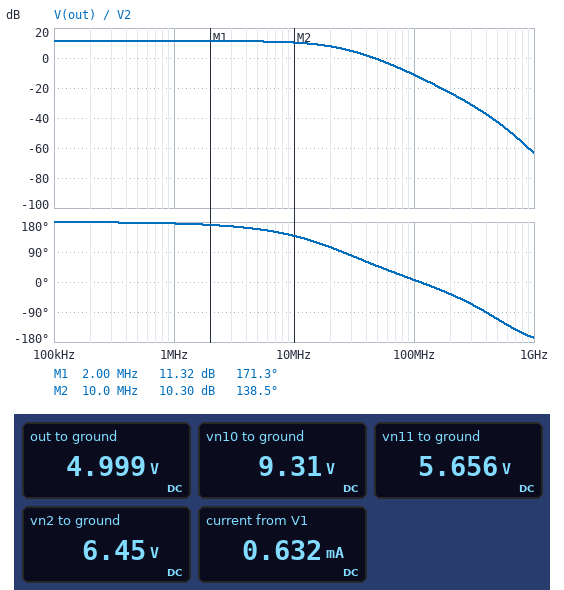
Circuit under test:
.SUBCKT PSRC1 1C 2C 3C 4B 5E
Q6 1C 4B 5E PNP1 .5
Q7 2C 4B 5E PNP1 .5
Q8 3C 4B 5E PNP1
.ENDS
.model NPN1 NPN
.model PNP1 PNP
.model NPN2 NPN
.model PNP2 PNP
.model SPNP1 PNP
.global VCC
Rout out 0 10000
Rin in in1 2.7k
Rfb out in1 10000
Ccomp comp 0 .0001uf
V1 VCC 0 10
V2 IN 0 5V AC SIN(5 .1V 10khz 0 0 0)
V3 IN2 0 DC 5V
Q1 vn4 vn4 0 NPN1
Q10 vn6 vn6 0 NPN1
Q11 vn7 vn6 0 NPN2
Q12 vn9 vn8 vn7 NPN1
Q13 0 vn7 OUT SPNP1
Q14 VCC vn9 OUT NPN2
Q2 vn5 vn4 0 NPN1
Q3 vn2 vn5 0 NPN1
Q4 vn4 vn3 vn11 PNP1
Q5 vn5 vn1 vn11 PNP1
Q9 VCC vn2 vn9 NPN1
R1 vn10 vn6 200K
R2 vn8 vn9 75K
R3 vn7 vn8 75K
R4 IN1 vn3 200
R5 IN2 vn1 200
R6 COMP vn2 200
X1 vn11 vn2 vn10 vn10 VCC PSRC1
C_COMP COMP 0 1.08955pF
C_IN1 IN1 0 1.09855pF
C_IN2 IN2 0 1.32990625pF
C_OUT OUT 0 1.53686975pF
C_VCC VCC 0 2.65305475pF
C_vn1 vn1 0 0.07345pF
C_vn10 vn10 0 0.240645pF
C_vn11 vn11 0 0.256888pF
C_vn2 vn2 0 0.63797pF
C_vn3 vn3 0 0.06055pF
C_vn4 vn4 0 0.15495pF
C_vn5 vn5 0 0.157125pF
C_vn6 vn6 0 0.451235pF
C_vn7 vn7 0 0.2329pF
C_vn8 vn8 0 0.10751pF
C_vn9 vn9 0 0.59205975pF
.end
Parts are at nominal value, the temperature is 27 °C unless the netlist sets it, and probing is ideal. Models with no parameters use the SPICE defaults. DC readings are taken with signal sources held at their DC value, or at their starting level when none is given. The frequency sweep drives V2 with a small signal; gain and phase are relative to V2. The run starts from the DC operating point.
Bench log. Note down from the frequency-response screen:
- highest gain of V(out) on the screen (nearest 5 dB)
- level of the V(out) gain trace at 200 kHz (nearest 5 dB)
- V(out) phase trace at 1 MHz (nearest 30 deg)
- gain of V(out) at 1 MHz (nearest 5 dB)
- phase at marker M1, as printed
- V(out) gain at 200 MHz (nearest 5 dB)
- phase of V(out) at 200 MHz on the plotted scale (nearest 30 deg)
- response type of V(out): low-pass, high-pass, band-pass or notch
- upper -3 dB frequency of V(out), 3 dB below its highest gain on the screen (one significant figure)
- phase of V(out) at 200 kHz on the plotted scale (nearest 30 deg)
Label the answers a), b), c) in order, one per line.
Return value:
a) 10 dB
b) 10 dB
c) 180 deg
d) 10 dB
e) 171.3 deg
f) -25 dB
g) -30 deg
h) low-pass
i) 20 MHz
j) 180 deg
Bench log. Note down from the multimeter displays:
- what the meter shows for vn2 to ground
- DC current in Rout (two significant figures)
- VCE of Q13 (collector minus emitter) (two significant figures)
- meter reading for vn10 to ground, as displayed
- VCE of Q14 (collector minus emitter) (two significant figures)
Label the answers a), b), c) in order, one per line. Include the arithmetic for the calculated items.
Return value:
a) 6.45 V
b) (4.999 V) / 10 kΩ = 500 µA
c) 0 V - 4.999 V = -5.0 V
d) 9.31 V
e) 10 V - 4.999 V = 5.0 V
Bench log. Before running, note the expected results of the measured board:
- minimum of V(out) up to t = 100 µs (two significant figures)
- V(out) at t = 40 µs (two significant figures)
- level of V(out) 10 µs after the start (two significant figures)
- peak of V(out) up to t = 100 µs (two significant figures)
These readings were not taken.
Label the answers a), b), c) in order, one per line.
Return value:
a) 4.6 V
b) 4.8 V
c) 4.8 V
d) 5.4 V
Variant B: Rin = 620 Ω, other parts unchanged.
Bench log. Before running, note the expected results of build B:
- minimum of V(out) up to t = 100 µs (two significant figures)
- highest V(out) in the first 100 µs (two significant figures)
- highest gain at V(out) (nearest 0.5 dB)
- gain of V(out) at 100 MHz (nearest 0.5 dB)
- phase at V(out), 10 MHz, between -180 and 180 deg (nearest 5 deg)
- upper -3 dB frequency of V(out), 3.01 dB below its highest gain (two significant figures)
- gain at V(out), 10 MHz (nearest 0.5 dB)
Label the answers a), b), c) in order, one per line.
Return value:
a) 3.4 V
b) 6.6 V
c) 24.0 dB
d) -5.5 dB
e) 105 deg
f) 3.7 MHz
g) 15.0 dB
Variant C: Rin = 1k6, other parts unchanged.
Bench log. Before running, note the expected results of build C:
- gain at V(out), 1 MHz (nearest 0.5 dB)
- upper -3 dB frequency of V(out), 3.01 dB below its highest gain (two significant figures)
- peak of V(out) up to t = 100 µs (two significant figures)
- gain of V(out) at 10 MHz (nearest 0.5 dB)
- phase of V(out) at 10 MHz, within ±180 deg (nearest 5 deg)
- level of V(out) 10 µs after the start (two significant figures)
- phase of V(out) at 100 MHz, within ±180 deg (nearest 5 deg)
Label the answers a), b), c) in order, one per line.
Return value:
a) 16.0 dB
b) 9.9 MHz
c) 5.6 V
d) 13.0 dB
e) 125 deg
f) 4.6 V
g) 20 deg
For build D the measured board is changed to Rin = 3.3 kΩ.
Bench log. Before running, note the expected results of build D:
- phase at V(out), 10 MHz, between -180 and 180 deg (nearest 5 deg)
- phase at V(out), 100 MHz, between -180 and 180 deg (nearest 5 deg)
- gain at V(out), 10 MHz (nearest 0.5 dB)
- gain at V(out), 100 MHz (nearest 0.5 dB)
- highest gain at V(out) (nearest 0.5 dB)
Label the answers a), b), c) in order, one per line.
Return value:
a) 145 deg
b) 0 deg
c) 9.0 dB
d) -12.5 dB
e) 9.5 dB
